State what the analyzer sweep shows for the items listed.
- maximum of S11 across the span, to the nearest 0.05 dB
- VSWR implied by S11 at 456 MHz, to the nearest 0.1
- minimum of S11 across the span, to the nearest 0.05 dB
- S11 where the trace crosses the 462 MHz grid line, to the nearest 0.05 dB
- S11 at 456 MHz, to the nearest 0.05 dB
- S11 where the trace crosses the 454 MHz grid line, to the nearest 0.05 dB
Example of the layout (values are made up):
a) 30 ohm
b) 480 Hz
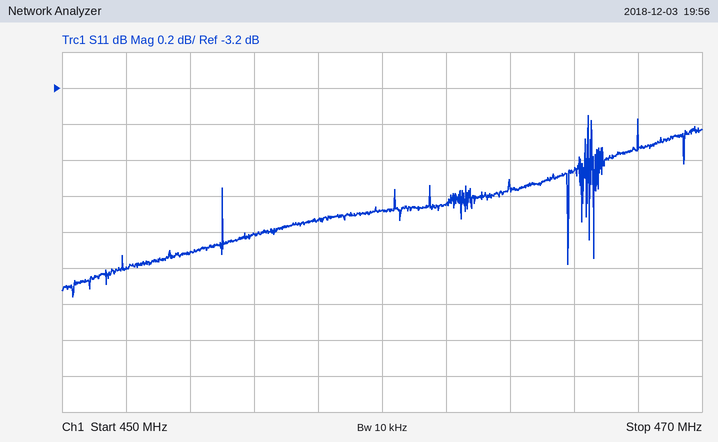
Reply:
a) -3.35 dB
b) 4.4
c) -4.35 dB
d) -3.85 dB
e) -4.00 dB
f) -4.10 dB
